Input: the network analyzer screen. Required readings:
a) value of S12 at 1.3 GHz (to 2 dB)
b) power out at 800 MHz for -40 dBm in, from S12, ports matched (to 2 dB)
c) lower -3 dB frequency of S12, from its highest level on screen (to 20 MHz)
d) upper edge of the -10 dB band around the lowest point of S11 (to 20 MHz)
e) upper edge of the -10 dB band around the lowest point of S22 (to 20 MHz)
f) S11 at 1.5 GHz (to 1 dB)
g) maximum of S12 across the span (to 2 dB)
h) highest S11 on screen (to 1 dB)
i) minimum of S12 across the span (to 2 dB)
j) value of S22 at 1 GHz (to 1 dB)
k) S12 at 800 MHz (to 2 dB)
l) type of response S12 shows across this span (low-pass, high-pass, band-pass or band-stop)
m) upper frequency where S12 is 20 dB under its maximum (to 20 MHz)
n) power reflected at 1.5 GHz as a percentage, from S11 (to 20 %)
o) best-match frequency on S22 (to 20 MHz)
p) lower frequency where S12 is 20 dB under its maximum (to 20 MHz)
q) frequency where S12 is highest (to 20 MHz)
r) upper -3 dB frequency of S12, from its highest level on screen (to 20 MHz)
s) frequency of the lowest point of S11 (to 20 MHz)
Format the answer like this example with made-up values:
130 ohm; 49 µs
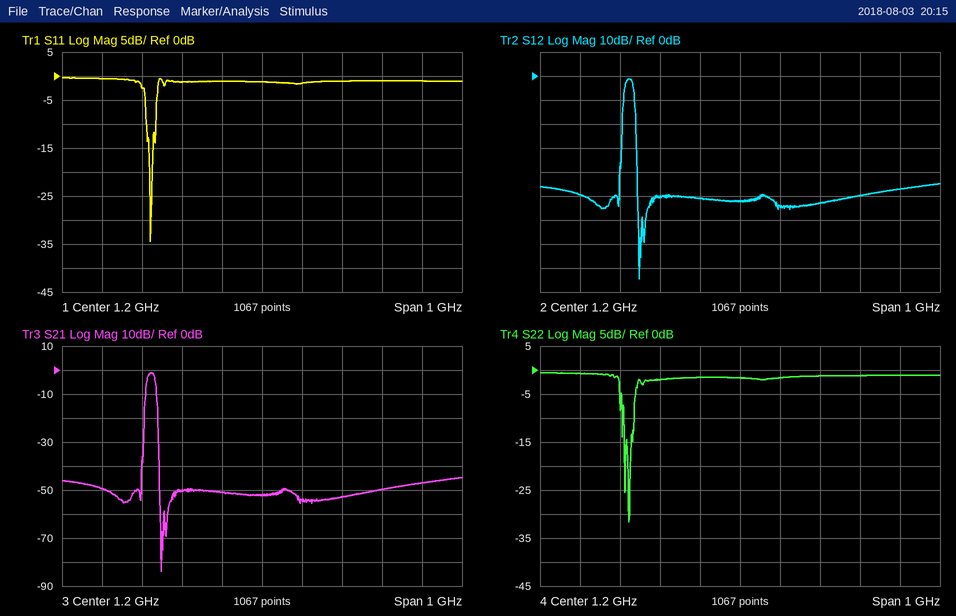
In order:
-54 dB; -90 dBm; 920 MHz; 940 MHz; 940 MHz; -1 dB; -2 dB; 0 dB; -84 dB; -2 dB; -50 dB; band-pass; 940 MHz; 80 %; 920 MHz; 900 MHz; 920 MHz; 940 MHz; 920 MHz
